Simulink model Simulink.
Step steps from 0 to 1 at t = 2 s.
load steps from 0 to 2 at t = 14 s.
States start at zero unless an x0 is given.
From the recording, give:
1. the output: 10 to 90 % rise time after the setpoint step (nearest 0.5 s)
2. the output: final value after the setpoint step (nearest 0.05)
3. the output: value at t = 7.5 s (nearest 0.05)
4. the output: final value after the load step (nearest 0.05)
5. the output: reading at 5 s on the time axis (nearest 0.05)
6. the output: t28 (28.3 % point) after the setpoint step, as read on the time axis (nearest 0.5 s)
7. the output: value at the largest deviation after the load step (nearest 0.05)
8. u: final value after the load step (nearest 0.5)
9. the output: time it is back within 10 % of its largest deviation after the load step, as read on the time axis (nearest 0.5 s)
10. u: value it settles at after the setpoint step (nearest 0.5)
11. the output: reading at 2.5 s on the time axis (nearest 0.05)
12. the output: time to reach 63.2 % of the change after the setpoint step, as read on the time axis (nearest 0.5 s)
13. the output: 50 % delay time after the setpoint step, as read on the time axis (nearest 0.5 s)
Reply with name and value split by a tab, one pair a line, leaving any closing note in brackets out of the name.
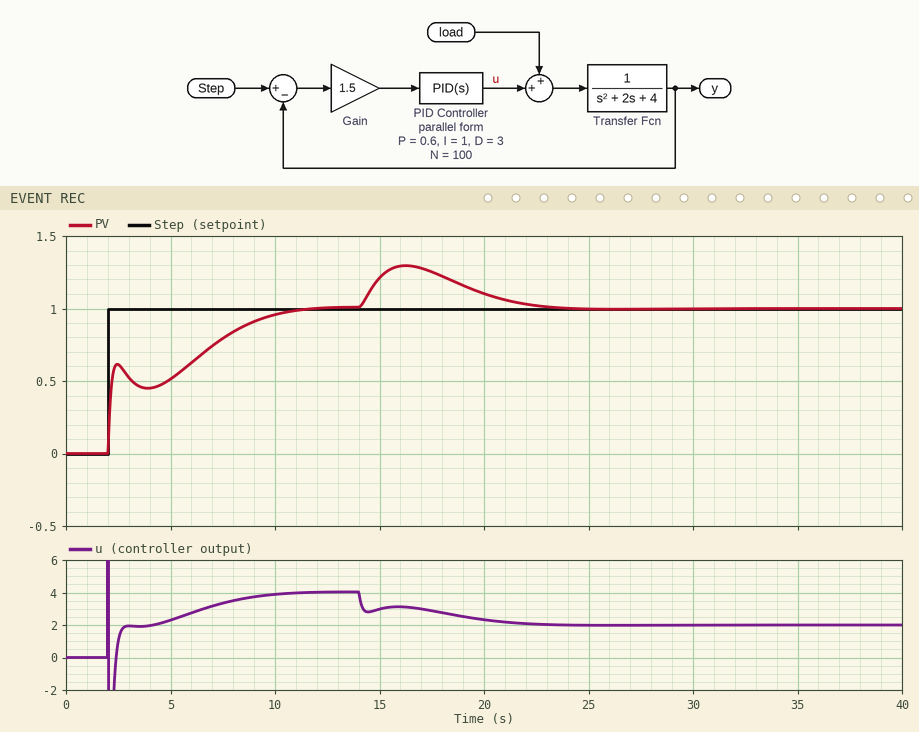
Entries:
the output: 10 to 90 % rise time after the setpoint step	7.0 s
the output: final value after the setpoint step	1.00
the output: value at t = 7.5 s	0.80
the output: final value after the load step	1.00
the output: reading at 5 s on the time axis	0.50
the output: t28 (28.3 % point) after the setpoint step, as read on the time axis	2.0 s
the output: value at the largest deviation after the load step	1.30
u: final value after the load step	2.0
the output: time it is back within 10 % of its largest deviation after the load step, as read on the time axis	22.0 s
u: value it settles at after the setpoint step	4.0
the output: reading at 2.5 s on the time axis	0.60
the output: time to reach 63.2 % of the change after the setpoint step, as read on the time axis	6.0 s
the output: 50 % delay time after the setpoint step, as read on the time axis	2.0 s
